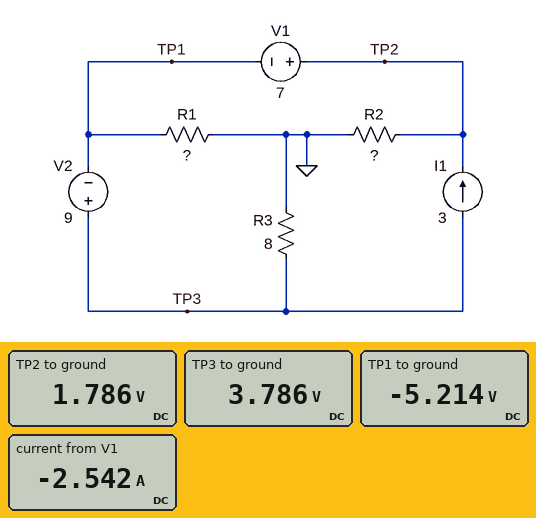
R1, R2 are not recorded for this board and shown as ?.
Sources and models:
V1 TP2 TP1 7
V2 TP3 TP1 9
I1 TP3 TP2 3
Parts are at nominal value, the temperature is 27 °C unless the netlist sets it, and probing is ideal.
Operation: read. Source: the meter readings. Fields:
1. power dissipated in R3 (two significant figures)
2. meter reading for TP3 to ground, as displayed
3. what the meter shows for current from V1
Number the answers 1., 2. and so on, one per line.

1. 1.8 W
2. 3.786 V
3. -2.542 A
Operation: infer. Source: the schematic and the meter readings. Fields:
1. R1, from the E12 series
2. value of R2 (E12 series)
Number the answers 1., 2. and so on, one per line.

1. 5.6 Ω
2. 3.9 Ω
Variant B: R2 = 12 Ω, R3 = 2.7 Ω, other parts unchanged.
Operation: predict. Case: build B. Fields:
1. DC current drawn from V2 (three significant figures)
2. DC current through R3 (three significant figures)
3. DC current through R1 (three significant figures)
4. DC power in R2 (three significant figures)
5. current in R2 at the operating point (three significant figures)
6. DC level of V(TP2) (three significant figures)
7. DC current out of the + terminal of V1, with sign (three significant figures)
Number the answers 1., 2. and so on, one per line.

1. 4.04 A
2. 1.04 A
3. 1.11 A
4. 54.1 mW
5. 67.1 mA
6. 805 mV
7. -2.93 A
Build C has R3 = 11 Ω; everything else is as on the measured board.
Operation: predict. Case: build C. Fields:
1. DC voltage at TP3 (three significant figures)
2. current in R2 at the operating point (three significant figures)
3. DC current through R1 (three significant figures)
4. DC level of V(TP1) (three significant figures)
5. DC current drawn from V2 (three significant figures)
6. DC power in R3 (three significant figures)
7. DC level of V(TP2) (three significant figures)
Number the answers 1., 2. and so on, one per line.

1. 4.03 V
2. 521 mA
3. 887 mA
4. -4.97 V
5. 3.37 A
6. 1.48 W
7. 2.03 V
